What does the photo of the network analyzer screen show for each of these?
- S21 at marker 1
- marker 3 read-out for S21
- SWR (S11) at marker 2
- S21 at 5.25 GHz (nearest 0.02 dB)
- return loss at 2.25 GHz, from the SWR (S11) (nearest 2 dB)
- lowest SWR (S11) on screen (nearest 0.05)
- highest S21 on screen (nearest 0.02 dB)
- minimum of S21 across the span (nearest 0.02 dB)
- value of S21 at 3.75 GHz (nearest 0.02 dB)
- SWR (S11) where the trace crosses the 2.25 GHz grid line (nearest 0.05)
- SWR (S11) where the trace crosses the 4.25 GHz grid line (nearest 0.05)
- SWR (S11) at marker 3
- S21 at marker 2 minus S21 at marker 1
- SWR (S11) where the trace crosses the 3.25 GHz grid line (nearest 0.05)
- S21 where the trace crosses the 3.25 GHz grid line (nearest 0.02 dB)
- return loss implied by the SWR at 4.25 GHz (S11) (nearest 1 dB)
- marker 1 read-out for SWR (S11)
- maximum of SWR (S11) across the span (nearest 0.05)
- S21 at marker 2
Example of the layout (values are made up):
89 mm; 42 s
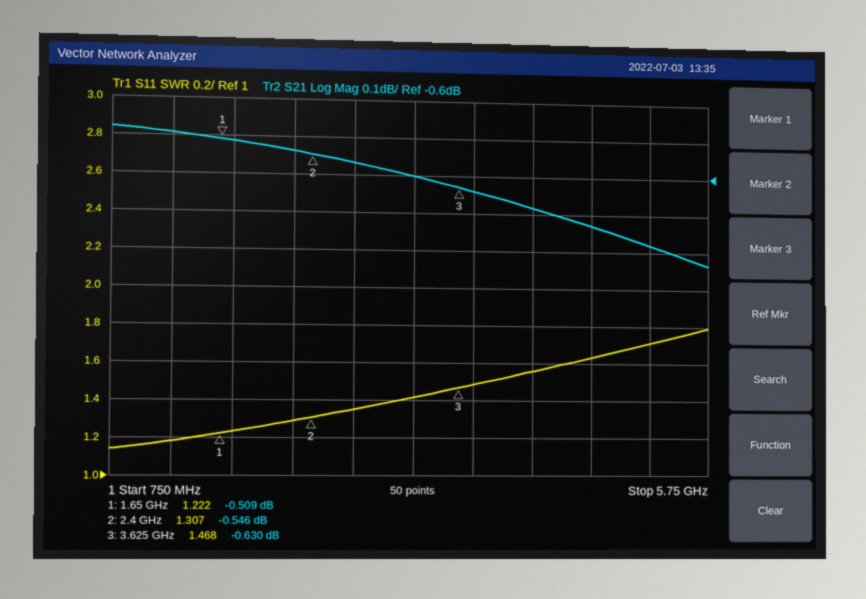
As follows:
-0.509 dB; -0.630 dB; 1.307; -0.78 dB; 18 dB; 1.15; -0.48 dB; -0.84 dB; -0.64 dB; 1.30; 1.55; 1.468; -0.037 dB; 1.40; -0.60 dB; 13 dB; 1.222; 1.80; -0.546 dB
